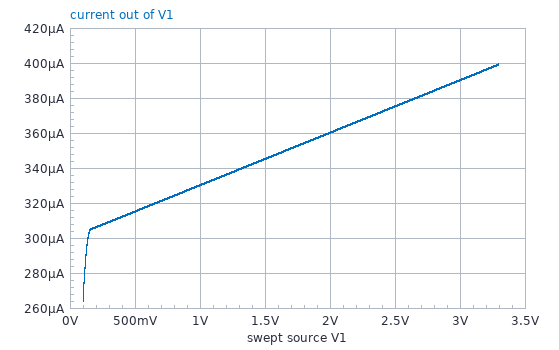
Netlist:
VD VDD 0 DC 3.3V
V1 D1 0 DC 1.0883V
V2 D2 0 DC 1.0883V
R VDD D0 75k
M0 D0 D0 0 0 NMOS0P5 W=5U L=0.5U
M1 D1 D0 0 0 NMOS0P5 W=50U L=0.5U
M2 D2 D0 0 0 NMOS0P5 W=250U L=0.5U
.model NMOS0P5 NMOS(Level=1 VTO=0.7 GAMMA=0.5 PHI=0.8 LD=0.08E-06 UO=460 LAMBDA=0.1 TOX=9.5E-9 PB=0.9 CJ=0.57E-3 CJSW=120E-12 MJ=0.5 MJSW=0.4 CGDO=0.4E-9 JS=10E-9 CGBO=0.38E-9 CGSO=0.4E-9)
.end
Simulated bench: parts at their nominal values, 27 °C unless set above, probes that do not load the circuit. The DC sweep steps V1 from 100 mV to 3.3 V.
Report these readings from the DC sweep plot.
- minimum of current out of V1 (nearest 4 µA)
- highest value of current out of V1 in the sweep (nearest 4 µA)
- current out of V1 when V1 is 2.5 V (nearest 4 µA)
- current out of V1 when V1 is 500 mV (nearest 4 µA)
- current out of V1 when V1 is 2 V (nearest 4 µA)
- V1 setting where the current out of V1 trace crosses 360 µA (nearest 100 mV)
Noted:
264 µA
400 µA
376 µA
316 µA
360 µA
2.0 V
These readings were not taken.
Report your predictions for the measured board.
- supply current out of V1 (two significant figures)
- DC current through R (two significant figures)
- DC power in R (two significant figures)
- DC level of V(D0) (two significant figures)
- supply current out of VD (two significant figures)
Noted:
330 µA
33 µA
80 µW
860 mV
33 µA
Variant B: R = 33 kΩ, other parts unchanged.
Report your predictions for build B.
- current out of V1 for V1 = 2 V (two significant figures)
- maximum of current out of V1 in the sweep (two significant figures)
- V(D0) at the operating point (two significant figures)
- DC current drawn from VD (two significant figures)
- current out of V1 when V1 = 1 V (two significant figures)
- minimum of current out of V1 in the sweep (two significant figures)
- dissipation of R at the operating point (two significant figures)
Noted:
790 µA
870 µA
930 mV
72 µA
720 µA
450 µA
170 µW
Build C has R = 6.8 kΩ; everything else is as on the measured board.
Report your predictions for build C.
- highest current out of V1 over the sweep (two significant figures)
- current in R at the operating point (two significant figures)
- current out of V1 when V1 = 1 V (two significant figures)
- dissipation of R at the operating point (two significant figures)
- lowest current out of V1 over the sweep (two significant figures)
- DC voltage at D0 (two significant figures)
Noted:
3.7 mA
310 µA
3.1 mA
660 µW
1.1 mA
1.2 V
